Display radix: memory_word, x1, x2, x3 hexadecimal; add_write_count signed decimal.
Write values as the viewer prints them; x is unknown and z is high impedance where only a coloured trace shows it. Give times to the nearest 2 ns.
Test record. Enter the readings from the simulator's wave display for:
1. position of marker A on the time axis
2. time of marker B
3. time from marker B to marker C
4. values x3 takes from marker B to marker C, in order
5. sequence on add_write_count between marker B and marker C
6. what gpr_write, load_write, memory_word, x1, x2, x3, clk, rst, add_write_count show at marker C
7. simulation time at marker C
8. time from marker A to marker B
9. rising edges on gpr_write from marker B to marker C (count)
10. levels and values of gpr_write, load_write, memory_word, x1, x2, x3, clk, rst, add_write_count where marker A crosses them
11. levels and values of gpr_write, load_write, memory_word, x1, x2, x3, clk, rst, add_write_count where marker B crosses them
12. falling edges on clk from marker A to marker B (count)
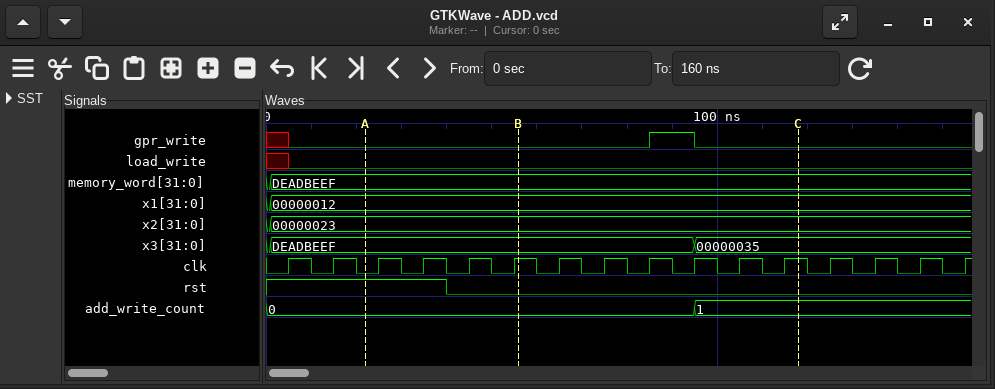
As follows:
22 ns
56 ns
62 ns
DEADBEEF, 00000035
0, 1
gpr_write=0, load_write=0, memory_word=DEADBEEF, x1=00000012, x2=00000023, x3=00000035, clk=1, rst=0, add_write_count=1
118 ns
34 ns
1
gpr_write=0, load_write=0, memory_word=DEADBEEF, x1=00000012, x2=00000023, x3=DEADBEEF, clk=0, rst=1, add_write_count=0
gpr_write=0, load_write=0, memory_word=DEADBEEF, x1=00000012, x2=00000023, x3=DEADBEEF, clk=1, rst=0, add_write_count=0
3
